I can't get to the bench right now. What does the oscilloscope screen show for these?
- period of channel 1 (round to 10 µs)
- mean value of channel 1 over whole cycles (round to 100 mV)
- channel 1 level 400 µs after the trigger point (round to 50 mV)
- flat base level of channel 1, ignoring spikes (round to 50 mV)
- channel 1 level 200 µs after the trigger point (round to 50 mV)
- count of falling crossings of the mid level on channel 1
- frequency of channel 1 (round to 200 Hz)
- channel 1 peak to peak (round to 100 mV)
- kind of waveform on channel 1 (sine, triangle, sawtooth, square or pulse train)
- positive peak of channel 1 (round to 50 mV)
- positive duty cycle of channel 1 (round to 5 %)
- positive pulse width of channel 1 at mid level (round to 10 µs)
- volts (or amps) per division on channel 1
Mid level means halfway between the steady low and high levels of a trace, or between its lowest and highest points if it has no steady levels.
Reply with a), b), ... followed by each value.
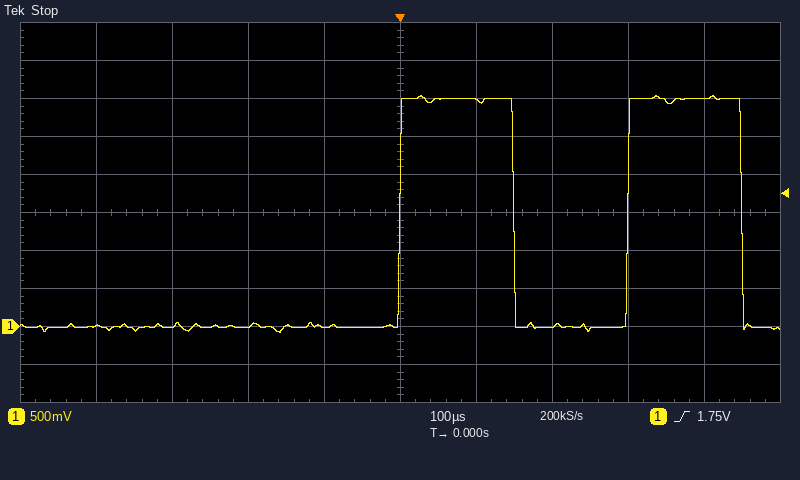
a) 300 µs
b) 1.5 V
c) 3.00 V
d) 0 mV
e) 0 mV
f) 2
g) 3.4 kHz
h) 3.10 V
i) square
j) 3.05 V
k) 50 %
l) 150 µs
m) 500 mV
